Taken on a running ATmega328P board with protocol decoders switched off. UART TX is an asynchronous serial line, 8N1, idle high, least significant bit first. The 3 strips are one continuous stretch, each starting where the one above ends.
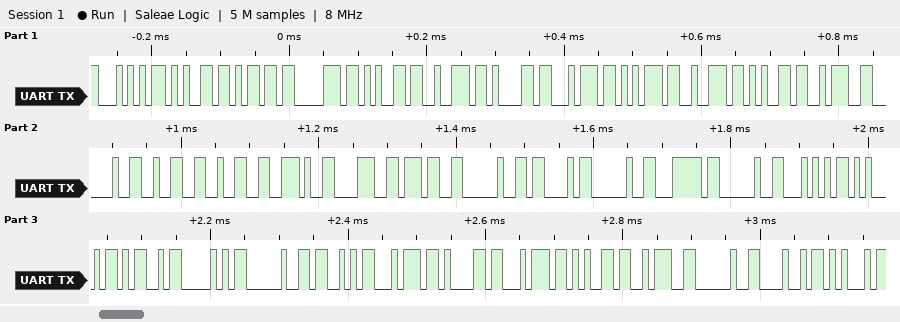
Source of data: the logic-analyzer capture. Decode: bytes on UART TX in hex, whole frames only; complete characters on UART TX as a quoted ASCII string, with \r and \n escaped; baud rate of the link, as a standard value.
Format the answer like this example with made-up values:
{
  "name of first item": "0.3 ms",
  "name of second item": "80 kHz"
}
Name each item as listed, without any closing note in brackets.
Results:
{
  "bytes on UART TX in hex, whole frames only": "54 65 6D 70 65 72 61 74 75 72 65 3A 20 32 32 2E 38 37 20 43 20 7C 20 54 45 4D 50 20 53 74 61 74 65 3A 20 48 45",
  "complete characters on UART TX as a quoted ASCII string, with \\r and \\n escaped": "\"Temperature: 22.87 C | TEMP State: HE\"",
  "baud rate of the link, as a standard value": "115200 baud"
}
